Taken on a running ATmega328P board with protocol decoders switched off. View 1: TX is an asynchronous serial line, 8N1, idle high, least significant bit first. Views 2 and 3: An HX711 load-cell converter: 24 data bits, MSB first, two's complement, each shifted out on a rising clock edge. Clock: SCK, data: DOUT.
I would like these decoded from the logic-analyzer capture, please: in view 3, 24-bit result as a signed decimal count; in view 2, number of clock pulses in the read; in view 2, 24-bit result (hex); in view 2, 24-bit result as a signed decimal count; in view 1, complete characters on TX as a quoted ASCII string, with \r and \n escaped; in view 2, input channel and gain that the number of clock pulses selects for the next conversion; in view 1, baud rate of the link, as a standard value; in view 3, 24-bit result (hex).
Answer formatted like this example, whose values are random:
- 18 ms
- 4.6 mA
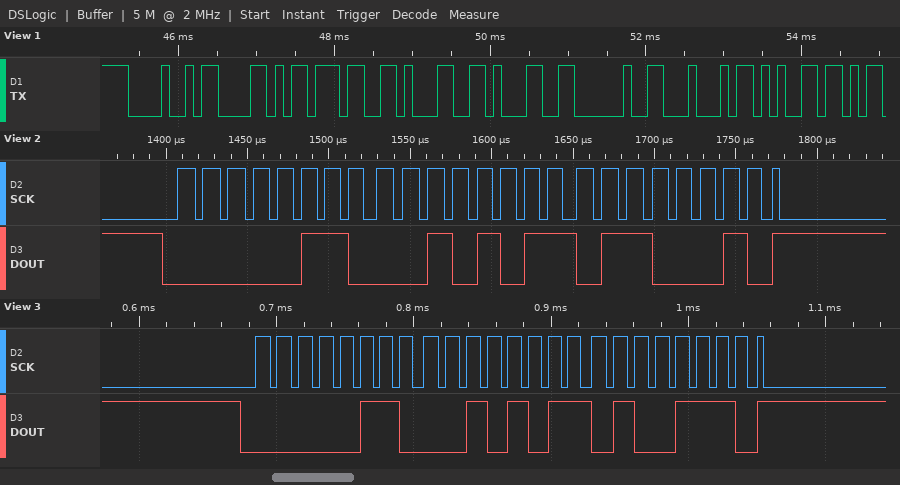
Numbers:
- 404302
- 25
- 0x062B62
- 404322
- "HX711 De"
- channel A, gain 128
- 9600 baud
- 0x062B4E
